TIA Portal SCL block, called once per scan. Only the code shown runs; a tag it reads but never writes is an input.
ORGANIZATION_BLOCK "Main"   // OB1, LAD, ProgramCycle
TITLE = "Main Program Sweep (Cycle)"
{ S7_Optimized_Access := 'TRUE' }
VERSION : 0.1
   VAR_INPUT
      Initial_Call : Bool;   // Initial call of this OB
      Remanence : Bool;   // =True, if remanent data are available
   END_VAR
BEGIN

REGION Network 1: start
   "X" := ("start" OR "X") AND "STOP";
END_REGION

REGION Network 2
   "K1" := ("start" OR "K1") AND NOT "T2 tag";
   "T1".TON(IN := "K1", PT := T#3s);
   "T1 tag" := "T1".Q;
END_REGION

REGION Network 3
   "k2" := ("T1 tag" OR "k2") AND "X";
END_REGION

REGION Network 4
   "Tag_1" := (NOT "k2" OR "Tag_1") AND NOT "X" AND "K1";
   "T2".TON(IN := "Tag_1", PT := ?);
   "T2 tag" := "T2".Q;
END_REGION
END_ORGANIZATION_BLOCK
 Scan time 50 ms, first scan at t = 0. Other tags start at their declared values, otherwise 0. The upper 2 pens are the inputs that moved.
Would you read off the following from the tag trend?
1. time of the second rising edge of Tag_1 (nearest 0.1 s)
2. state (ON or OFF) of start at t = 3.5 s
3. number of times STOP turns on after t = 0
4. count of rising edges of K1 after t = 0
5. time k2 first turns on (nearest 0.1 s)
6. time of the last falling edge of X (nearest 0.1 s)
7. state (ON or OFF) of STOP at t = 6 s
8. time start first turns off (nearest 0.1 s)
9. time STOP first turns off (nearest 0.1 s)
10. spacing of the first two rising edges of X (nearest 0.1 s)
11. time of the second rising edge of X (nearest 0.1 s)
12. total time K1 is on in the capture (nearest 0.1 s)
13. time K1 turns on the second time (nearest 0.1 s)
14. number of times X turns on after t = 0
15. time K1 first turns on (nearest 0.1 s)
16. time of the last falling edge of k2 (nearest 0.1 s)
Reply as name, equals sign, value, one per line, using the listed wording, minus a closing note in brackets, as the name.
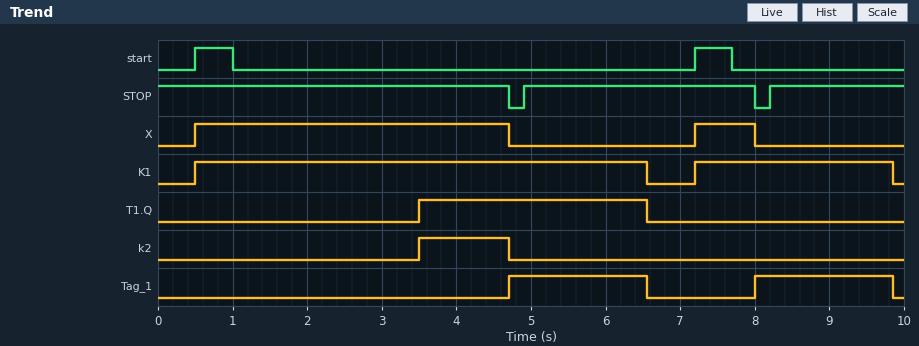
time of the second rising edge of Tag_1 = 8.0 s
state (ON or OFF) of start at t = 3.5 s = OFF
number of times STOP turns on after t = 0 = 2
count of rising edges of K1 after t = 0 = 2
time k2 first turns on = 3.5 s
time of the last falling edge of X = 8.0 s
state (ON or OFF) of STOP at t = 6 s = ON
time start first turns off = 1.0 s
time STOP first turns off = 4.7 s
spacing of the first two rising edges of X = 6.7 s
time of the second rising edge of X = 7.2 s
total time K1 is on in the capture = 8.7 s
time K1 turns on the second time = 7.2 s
number of times X turns on after t = 0 = 2
time K1 first turns on = 0.5 s
time of the last falling edge of k2 = 4.7 s
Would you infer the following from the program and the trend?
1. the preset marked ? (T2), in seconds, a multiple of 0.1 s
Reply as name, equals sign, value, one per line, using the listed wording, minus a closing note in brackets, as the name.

the preset marked ? (T2), in seconds, a multiple of 0.1 s = 1.8 s
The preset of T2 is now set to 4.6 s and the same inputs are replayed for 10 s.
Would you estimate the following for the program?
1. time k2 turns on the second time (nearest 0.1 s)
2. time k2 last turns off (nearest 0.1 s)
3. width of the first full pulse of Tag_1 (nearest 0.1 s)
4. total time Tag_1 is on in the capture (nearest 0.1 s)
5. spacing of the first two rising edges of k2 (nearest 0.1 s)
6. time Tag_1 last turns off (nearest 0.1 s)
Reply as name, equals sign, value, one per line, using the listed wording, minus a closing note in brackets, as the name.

time k2 turns on the second time = 7.2 s
time k2 last turns off = 8.0 s
width of the first full pulse of Tag_1 = 2.5 s
total time Tag_1 is on in the capture = 4.5 s
spacing of the first two rising edges of k2 = 3.7 s
time Tag_1 last turns off = 7.2 s
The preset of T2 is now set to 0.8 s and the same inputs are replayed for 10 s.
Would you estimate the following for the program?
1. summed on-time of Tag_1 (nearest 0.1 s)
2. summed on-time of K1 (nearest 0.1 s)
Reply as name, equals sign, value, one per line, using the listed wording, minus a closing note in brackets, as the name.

summed on-time of Tag_1 = 1.7 s
summed on-time of K1 = 6.7 s
